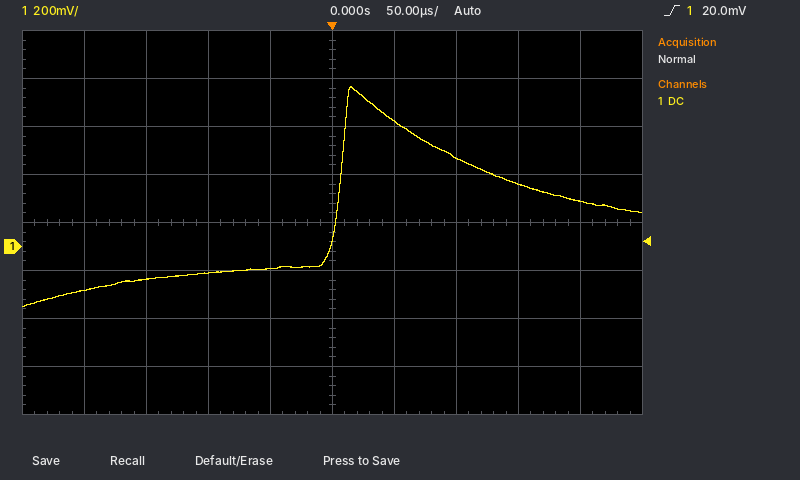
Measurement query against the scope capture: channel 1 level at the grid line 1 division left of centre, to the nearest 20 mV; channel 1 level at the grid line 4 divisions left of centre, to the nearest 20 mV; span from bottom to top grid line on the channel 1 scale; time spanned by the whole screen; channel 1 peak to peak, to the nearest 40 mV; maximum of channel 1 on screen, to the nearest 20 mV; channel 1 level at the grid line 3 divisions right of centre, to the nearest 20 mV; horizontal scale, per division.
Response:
-100 mV
-180 mV
1.6 V
500 µs
920 mV
660 mV
260 mV
50 µs
